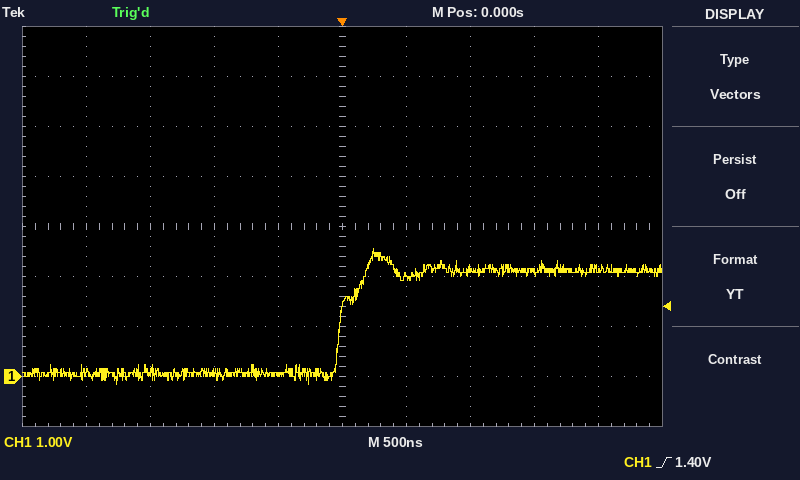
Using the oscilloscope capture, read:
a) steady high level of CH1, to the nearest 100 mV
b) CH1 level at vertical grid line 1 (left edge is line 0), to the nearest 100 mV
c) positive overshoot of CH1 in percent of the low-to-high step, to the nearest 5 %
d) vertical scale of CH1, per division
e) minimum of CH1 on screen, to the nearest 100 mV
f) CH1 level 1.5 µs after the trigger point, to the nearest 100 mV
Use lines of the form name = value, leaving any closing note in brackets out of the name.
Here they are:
steady high level of CH1, to the nearest 100 mV = 2.1 V
CH1 level at vertical grid line 1 (left edge is line 0), to the nearest 100 mV = 100 mV
positive overshoot of CH1 in percent of the low-to-high step, to the nearest 5 % = 20 %
vertical scale of CH1, per division = 1 V
minimum of CH1 on screen, to the nearest 100 mV = -200 mV
CH1 level 1.5 µs after the trigger point, to the nearest 100 mV = 2.1 V
